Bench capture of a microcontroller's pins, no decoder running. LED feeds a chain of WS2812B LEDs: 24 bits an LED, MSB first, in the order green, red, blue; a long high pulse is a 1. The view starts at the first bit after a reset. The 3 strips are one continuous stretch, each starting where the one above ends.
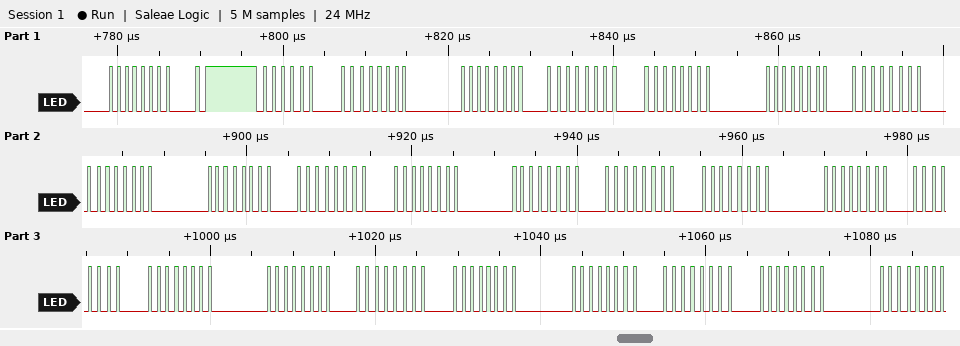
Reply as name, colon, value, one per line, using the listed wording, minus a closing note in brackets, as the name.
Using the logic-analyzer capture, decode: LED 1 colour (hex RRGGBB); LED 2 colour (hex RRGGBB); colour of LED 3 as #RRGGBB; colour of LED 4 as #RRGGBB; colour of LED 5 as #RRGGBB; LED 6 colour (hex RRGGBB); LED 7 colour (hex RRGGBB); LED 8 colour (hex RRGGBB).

LED 1 colour: #400000
LED 2 colour: #000000
colour of LED 3 as #RRGGBB: #000000
colour of LED 4 as #RRGGBB: #000000
colour of LED 5 as #RRGGBB: #000000
LED 6 colour: #000000
LED 7 colour: #000000
LED 8 colour: #000000
